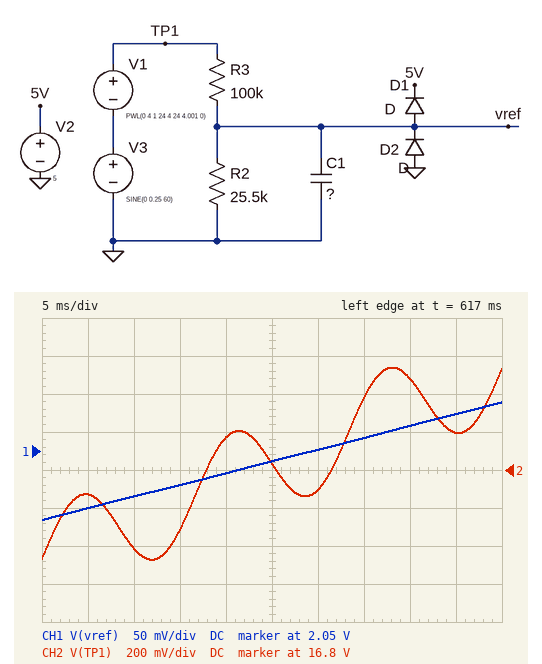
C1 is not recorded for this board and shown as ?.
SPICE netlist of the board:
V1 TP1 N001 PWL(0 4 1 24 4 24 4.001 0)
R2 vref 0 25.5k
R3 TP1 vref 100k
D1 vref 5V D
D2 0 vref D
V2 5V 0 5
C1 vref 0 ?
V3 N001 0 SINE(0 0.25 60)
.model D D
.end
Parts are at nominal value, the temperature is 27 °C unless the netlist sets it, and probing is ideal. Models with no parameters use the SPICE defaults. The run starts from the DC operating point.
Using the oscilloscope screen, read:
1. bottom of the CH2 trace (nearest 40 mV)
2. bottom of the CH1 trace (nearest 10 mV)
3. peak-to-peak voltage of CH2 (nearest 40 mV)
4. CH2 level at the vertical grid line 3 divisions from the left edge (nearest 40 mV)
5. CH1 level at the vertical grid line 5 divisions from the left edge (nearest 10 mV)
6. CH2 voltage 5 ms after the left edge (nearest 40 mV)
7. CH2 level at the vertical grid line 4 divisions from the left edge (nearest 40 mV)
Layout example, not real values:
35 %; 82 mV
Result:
16.32 V; 1.96 V; 1.00 V; 16.48 V; 2.04 V; 16.68 V; 16.96 V
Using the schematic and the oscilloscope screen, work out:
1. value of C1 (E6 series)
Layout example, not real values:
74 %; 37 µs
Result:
22 µF
